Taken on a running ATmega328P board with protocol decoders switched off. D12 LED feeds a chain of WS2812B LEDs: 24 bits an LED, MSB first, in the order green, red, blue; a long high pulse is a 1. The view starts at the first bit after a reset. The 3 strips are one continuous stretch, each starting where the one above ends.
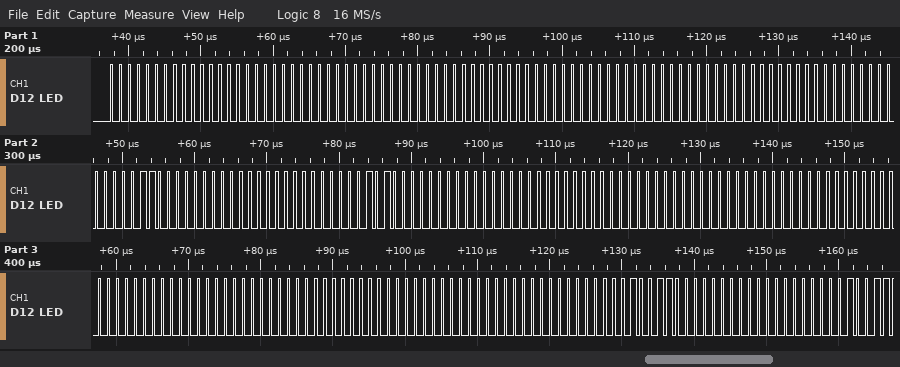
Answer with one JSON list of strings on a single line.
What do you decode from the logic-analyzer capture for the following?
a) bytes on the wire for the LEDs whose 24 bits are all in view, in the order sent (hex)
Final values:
["00 00 00 00 00 00 00 00 00 00 00 0C 00 00 05 00 00 00 00 00 00 00 00 00 00 00 00 00 00 13 00 00 13"]
